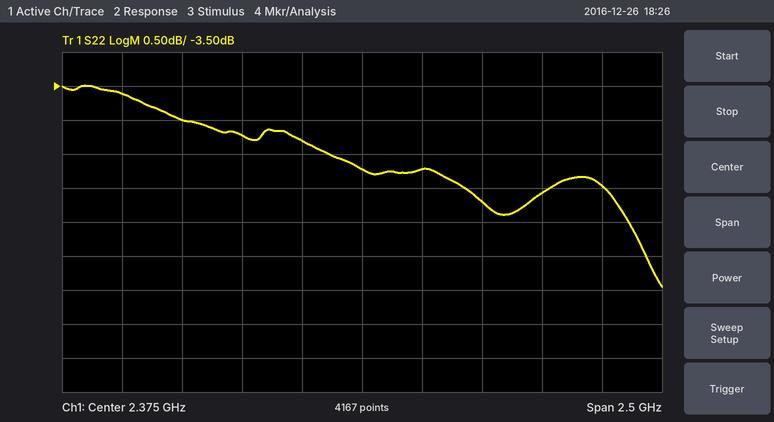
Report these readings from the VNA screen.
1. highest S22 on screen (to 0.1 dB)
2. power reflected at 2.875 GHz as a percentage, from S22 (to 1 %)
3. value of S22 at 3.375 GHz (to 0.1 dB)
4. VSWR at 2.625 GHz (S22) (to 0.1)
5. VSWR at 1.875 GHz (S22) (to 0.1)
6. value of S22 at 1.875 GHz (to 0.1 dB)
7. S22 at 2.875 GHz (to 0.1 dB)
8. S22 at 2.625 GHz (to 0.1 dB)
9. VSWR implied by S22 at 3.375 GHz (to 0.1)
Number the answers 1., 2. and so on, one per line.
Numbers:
1. -3.5 dB
2. 30 %
3. -5.0 dB
4. 3.8
5. 4.2
6. -4.2 dB
7. -5.2 dB
8. -4.7 dB
9. 3.6
